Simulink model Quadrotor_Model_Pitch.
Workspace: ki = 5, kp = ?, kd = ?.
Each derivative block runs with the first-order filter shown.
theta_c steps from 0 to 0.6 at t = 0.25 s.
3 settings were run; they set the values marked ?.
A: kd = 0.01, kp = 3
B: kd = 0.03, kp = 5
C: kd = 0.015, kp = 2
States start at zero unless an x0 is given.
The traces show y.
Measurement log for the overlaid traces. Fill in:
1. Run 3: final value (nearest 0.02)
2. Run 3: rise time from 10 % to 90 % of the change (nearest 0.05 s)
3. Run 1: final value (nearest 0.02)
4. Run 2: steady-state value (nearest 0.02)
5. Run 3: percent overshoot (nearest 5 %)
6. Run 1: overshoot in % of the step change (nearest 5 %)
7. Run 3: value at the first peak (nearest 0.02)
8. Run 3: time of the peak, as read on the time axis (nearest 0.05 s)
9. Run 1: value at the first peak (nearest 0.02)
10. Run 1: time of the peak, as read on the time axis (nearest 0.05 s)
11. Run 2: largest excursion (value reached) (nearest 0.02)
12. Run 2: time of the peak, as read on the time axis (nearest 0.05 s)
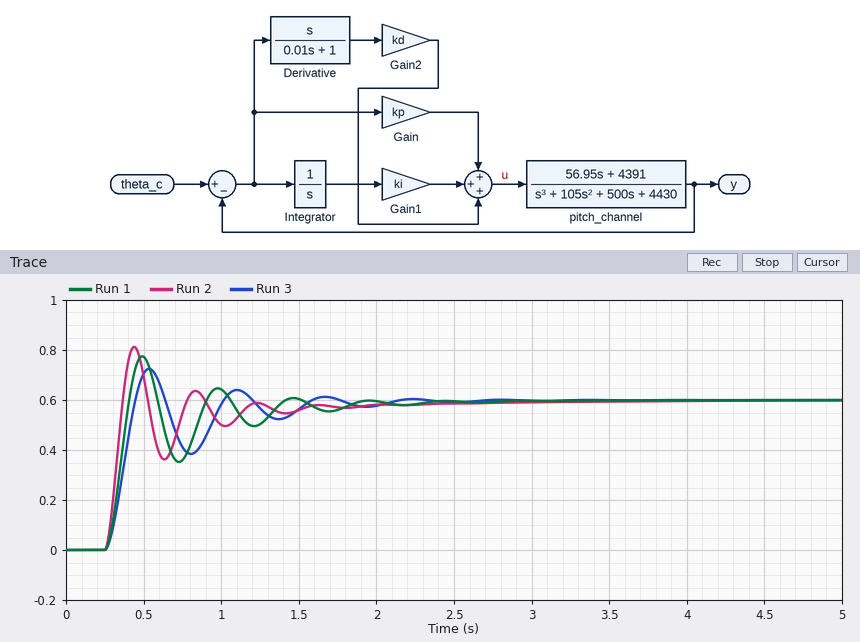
0.60
0.15 s
0.60
0.60
20 %
30 %
0.72
0.55 s
0.78
0.50 s
0.82
0.45 s
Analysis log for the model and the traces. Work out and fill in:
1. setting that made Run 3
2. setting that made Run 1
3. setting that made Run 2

C
A
B
